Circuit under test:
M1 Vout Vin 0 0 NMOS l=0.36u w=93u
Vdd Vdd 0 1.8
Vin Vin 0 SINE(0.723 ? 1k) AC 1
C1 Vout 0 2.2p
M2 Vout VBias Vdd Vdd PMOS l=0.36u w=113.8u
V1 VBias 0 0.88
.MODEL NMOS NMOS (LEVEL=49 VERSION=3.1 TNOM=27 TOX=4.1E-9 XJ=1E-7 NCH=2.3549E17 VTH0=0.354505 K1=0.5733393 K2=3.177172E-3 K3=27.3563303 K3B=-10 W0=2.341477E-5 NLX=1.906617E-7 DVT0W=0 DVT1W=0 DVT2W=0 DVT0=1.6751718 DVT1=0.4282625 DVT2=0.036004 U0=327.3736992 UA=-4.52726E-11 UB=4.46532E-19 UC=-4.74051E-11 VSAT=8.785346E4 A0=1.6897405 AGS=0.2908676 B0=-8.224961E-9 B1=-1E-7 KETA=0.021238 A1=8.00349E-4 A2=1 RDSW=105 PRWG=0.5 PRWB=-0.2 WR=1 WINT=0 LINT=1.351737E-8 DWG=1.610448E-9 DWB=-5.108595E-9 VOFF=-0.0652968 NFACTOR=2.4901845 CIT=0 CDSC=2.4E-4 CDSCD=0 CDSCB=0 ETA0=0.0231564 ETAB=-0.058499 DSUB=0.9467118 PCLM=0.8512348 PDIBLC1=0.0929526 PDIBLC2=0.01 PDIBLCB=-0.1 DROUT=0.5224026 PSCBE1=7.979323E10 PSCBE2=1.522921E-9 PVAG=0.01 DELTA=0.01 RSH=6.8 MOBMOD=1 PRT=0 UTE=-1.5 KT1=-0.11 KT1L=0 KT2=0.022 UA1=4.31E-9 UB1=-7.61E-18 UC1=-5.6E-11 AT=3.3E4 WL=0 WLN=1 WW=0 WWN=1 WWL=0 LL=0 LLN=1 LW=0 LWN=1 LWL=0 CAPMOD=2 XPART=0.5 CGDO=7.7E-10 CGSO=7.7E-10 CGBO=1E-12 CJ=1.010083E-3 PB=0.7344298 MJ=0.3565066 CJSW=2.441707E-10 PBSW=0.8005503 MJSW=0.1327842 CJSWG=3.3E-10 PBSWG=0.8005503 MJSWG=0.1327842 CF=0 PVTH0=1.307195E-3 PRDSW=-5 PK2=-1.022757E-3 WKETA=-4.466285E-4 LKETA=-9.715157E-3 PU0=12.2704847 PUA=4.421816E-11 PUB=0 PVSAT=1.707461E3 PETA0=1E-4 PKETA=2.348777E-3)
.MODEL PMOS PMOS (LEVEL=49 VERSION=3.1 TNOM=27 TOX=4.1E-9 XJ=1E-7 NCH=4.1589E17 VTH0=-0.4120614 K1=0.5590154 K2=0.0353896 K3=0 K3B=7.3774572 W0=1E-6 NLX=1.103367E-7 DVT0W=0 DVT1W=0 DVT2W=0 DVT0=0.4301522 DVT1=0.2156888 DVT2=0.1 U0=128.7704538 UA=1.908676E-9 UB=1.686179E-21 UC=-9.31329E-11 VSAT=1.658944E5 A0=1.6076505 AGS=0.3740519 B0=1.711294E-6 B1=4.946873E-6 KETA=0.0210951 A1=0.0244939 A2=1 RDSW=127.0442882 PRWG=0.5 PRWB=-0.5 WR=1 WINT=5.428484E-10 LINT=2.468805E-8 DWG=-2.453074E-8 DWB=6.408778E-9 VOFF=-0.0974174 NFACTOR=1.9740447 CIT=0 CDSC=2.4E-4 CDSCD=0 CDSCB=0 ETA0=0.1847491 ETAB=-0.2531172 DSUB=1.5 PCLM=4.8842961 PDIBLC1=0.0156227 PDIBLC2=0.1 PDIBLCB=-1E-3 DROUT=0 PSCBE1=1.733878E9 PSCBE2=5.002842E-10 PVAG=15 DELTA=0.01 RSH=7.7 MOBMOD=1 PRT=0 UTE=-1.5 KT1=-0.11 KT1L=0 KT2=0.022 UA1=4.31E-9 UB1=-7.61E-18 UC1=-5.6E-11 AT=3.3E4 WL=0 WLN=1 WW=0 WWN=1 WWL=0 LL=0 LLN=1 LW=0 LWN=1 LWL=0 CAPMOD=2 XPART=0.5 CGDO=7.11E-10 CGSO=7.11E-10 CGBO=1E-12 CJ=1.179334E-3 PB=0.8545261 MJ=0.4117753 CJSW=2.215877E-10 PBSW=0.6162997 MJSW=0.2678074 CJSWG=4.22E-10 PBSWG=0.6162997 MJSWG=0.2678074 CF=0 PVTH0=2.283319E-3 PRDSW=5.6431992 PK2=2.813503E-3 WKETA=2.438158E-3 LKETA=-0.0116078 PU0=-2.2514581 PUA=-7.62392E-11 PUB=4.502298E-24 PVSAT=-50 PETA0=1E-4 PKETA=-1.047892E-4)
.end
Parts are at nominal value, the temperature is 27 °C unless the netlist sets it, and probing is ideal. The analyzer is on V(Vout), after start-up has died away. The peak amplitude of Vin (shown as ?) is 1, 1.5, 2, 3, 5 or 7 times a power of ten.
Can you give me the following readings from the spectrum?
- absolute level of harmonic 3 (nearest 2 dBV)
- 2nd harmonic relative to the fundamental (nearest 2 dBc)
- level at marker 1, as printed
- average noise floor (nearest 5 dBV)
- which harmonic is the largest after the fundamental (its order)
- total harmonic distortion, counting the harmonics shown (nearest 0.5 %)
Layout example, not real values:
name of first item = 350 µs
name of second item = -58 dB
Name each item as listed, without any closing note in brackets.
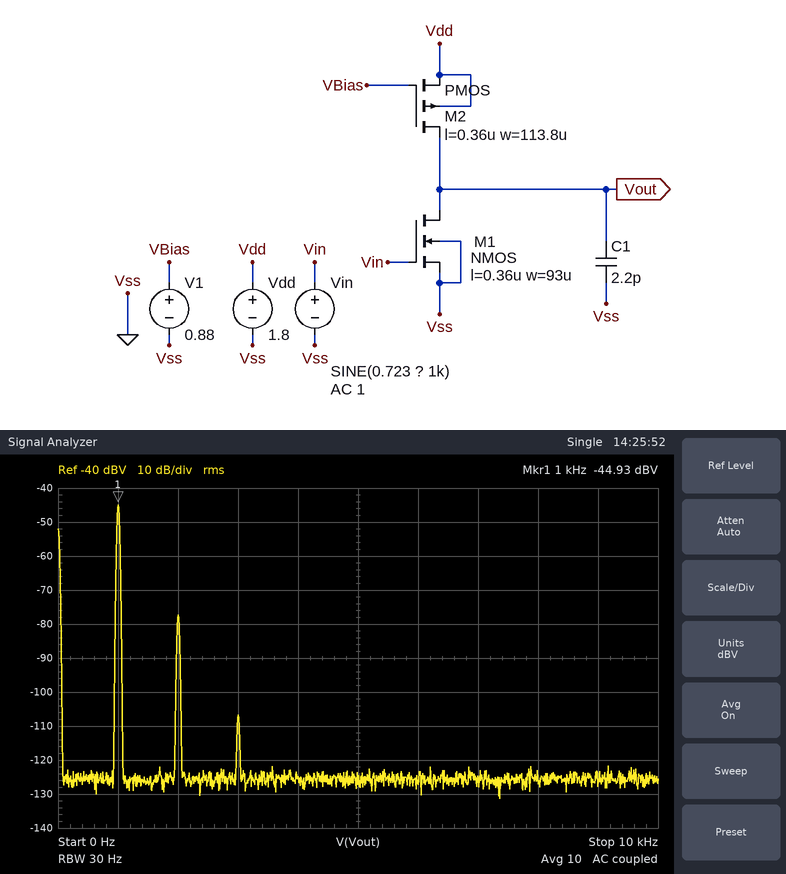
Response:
absolute level of harmonic 3 = -106 dBV
2nd harmonic relative to the fundamental = -32 dBc
level at marker 1, as printed = -44.93 dBV
average noise floor = -125 dBV
which harmonic is the largest after the fundamental = 2
total harmonic distortion, counting the harmonics shown = 2.5 %
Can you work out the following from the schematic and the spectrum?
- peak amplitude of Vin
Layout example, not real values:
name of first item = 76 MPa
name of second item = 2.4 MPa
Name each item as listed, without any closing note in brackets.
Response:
peak amplitude of Vin = 700 µV
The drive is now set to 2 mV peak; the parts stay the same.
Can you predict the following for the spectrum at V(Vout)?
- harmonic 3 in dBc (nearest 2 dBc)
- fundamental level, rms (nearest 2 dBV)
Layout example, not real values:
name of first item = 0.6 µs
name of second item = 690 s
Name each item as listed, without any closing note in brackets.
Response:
harmonic 3 in dBc = -44 dBc
fundamental level, rms = -36 dBV
